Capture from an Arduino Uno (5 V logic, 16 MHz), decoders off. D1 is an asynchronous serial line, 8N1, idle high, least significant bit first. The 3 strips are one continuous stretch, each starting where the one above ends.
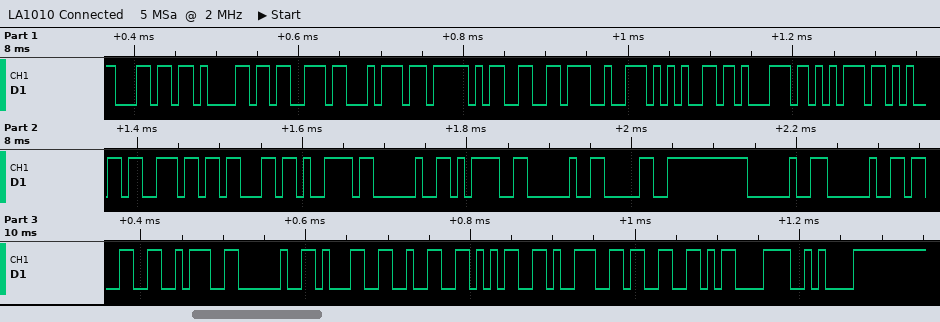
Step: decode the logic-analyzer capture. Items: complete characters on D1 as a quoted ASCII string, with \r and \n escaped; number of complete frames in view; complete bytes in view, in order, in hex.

"last_frequency = 0  3: 12593\r\n"
30
0x6C 0x61 0x73 0x74 0x5F 0x66 0x72 0x65 0x71 0x75 0x65 0x6E 0x63 0x79 0x20 0x3D 0x20 0x30 0x20 0x20 0x33 0x3A 0x20 0x31 0x32 0x35 0x39 0x33 0x0D 0x0A
